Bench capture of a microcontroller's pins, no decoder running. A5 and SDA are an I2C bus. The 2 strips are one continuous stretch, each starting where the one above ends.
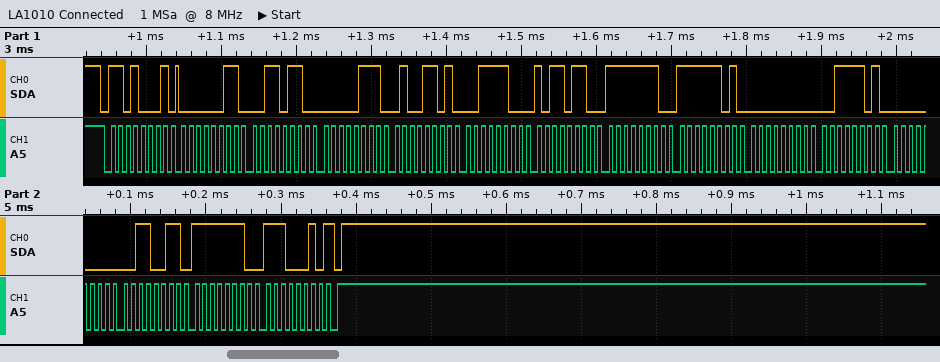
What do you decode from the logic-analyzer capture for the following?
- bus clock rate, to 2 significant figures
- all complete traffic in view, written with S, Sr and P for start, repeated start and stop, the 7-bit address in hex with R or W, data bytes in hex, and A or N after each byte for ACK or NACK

100 kHz
S 68R A 03 A 36 A 07 A 4D A 3C A B6 A FE A FD A 00 A 3D A 00 A 33 A FE A E2 N P
